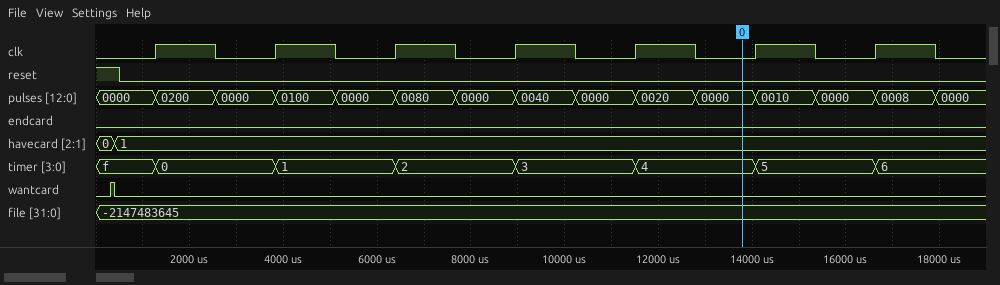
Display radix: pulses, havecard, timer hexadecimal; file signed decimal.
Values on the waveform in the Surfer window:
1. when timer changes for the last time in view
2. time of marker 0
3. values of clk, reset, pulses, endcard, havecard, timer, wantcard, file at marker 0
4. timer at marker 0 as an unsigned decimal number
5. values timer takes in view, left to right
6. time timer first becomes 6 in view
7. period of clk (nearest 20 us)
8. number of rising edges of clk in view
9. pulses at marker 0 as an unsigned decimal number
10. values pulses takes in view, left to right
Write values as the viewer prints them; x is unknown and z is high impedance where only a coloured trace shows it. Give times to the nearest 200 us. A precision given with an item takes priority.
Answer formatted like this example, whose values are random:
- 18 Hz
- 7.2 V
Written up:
- 16600 us
- 13800 us
- clk=0, reset=0, pulses=0000, endcard=0, havecard=1, timer=4, wantcard=0, file=-2147483645
- 4
- f, 0, 1, 2, 3, 4, 5, 6
- 16600 us
- 2560 us
- 7
- 0
- 0000, 0200, 0000, 0100, 0000, 0080, 0000, 0040, 0000, 0020, 0000, 0010, 0000, 0008, 0000
